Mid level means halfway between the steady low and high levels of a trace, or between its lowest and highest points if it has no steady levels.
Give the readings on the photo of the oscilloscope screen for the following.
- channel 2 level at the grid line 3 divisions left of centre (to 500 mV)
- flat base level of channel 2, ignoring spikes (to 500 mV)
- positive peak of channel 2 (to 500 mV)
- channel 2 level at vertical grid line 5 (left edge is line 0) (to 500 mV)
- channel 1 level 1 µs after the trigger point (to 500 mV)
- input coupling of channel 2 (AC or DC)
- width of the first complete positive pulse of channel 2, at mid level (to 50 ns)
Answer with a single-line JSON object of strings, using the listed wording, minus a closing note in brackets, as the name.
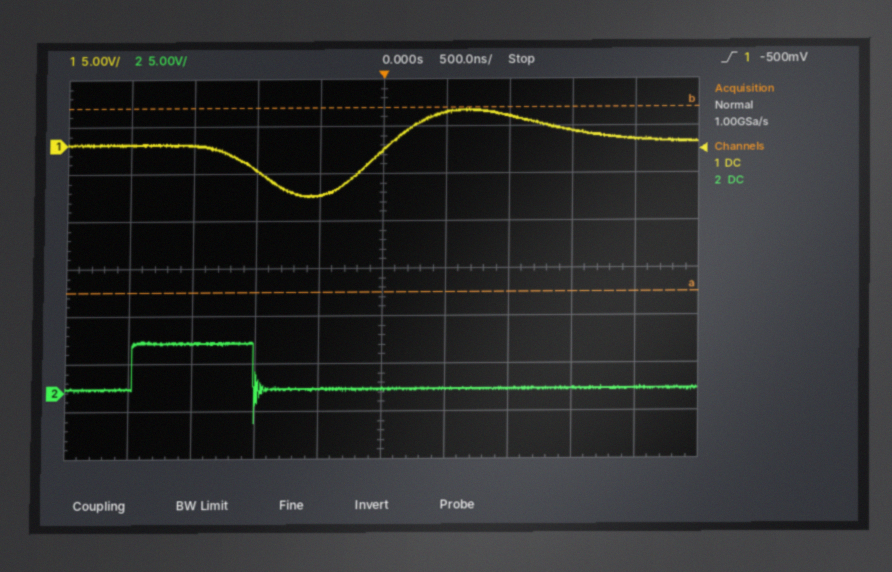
{"channel 2 level at the grid line 3 divisions left of centre": "5.0 V", "flat base level of channel 2, ignoring spikes": "500 mV", "positive peak of channel 2": "5.5 V", "channel 2 level at vertical grid line 5 (left edge is line 0)": "500 mV", "channel 1 level 1 µs after the trigger point": "3.0 V", "input coupling of channel 2": "DC", "width of the first complete positive pulse of channel 2, at mid level": "950 ns"}
